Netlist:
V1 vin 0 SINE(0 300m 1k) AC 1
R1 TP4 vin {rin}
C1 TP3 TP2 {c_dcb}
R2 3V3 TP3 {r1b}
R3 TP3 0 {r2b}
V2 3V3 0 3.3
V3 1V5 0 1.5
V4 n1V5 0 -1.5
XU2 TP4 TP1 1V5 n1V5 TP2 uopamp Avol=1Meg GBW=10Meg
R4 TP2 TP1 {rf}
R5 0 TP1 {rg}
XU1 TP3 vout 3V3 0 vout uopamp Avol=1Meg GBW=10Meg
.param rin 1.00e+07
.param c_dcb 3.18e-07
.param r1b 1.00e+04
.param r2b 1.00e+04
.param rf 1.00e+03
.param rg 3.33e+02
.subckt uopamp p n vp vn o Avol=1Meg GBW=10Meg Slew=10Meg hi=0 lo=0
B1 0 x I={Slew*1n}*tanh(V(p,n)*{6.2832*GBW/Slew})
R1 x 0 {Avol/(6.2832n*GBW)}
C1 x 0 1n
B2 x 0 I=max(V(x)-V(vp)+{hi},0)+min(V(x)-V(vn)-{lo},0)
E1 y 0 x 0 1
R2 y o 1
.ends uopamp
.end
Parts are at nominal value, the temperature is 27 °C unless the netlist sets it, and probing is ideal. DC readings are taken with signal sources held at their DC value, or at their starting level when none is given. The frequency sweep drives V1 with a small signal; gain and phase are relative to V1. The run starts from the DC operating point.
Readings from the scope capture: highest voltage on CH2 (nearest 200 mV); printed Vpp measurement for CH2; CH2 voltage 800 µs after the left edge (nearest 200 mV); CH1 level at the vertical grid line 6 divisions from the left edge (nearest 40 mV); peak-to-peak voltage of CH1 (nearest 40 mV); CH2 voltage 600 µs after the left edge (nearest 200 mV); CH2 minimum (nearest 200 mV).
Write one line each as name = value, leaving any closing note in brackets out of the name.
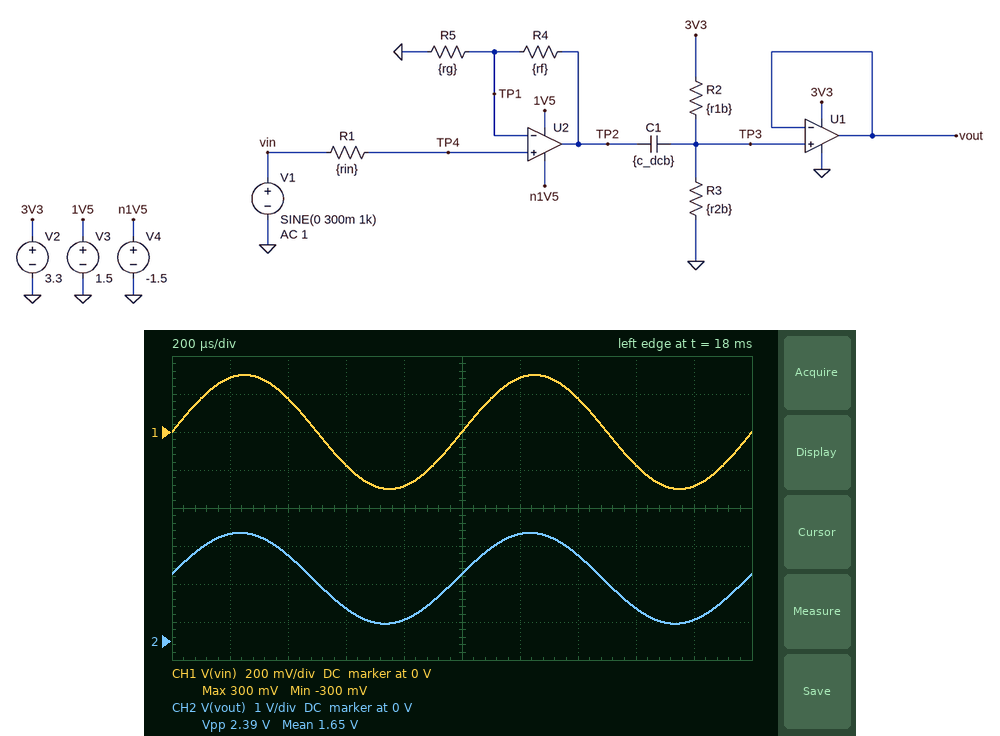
highest voltage on CH2 = 2.8 V
printed Vpp measurement for CH2 = 2.39 V
CH2 voltage 800 µs after the left edge = 600 mV
CH1 level at the vertical grid line 6 divisions from the left edge = 280 mV
peak-to-peak voltage of CH1 = 600 mV
CH2 voltage 600 µs after the left edge = 800 mV
CH2 minimum = 400 mV
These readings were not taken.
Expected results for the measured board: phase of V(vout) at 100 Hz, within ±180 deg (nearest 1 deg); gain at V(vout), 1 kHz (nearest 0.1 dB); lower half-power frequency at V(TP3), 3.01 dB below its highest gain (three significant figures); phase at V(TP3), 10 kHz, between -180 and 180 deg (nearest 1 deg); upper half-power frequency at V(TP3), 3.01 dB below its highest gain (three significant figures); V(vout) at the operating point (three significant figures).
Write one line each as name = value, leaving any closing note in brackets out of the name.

phase of V(vout) at 100 Hz, within ±180 deg = 45 deg
gain at V(vout), 1 kHz = 12.0 dB
lower half-power frequency at V(TP3), 3.01 dB below its highest gain = 100 Hz
phase at V(TP3), 10 kHz, between -180 and 180 deg = 0 deg
upper half-power frequency at V(TP3), 3.01 dB below its highest gain = 2.50 MHz
V(vout) at the operating point = 1.65 V
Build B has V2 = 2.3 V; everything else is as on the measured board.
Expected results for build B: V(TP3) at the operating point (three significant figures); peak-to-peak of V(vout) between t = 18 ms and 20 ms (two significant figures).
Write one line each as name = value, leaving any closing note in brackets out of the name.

V(TP3) at the operating point = 1.15 V
peak-to-peak of V(vout) between t = 18 ms and 20 ms = 2.3 V
